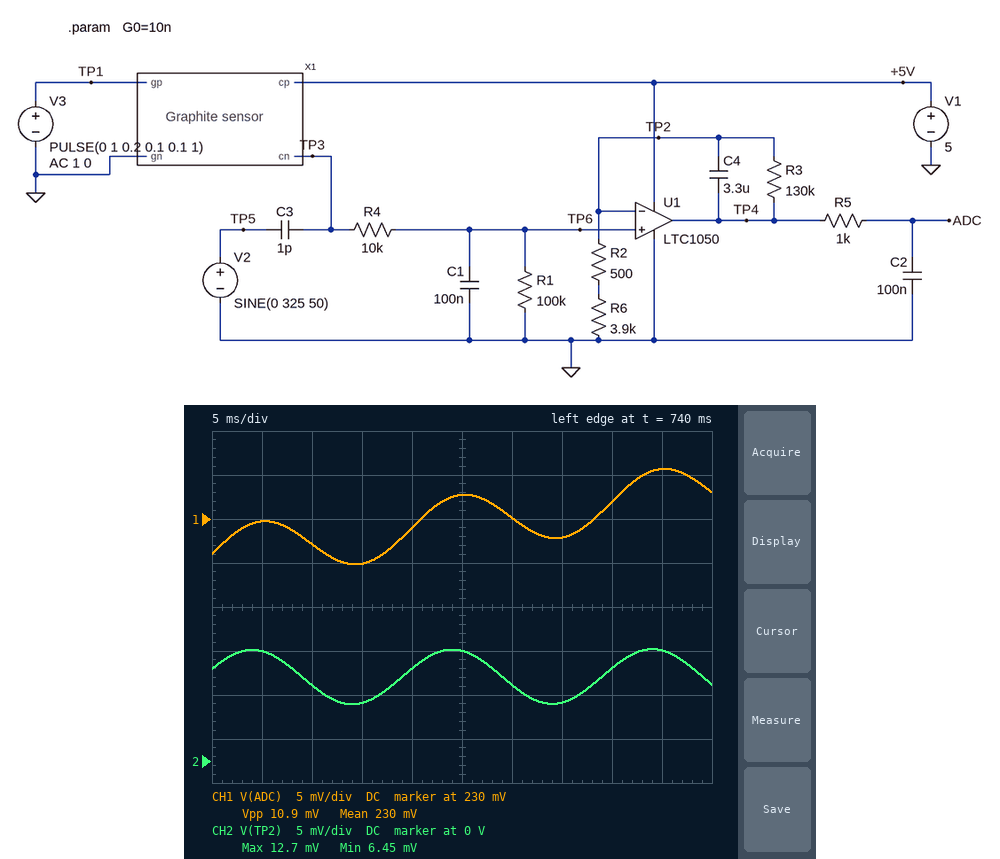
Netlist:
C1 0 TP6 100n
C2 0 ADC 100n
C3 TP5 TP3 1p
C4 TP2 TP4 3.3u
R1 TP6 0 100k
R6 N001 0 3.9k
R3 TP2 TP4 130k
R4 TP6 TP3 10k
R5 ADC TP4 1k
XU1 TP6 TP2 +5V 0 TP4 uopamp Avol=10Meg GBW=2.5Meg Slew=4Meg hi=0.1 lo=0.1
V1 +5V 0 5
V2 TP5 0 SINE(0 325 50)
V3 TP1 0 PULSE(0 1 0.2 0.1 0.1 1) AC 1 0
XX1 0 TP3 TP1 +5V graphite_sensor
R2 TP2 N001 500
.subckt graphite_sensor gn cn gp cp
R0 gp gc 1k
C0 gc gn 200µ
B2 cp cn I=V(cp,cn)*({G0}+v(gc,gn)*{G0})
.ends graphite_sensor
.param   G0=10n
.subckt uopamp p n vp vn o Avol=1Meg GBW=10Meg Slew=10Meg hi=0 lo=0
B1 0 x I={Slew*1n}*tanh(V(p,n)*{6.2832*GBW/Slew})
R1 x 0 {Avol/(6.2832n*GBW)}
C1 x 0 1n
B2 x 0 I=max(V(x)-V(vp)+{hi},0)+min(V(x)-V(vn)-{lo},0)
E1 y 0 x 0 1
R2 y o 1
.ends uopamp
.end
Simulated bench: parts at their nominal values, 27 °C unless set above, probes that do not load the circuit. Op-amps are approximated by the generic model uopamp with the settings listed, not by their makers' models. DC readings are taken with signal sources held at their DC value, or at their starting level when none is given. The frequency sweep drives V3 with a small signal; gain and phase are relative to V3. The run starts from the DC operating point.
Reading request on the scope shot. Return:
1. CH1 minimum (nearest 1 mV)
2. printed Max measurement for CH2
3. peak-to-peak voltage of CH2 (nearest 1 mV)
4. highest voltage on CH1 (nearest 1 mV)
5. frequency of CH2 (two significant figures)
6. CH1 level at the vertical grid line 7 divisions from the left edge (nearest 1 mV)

225 mV
12.7 mV
6 mV
236 mV
50 Hz
228 mV
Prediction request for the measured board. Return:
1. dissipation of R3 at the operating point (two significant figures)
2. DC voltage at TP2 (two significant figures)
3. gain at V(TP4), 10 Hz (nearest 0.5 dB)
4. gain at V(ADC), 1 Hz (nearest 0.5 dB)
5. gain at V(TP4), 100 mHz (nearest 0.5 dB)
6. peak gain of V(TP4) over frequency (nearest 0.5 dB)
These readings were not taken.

170 nW
5.0 mV
-66.0 dB
-29.5 dB
-16.5 dB
-16.5 dB
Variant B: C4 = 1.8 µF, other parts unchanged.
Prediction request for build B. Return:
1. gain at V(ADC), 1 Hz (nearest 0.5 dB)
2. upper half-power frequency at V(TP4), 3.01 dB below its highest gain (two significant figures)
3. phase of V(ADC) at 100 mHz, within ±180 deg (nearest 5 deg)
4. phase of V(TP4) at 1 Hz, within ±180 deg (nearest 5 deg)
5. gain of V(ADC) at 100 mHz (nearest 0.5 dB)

-25.5 dB
470 mHz
-15 deg
-110 deg
-16.5 dB
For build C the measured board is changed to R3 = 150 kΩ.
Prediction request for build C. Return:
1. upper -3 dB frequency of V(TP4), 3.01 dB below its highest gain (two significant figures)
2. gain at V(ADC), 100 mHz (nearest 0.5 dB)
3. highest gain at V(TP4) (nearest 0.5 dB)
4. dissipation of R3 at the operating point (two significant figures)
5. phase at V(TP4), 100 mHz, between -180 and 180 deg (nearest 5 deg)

280 mHz
-15.5 dB
-15.0 dB
190 nW
-25 deg
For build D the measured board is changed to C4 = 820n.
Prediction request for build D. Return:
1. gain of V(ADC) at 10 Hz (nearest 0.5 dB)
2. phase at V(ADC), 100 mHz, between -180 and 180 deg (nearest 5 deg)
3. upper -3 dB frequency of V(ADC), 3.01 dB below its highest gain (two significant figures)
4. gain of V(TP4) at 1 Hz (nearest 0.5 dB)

-56.0 dB
-10 deg
650 mHz
-22.0 dB
